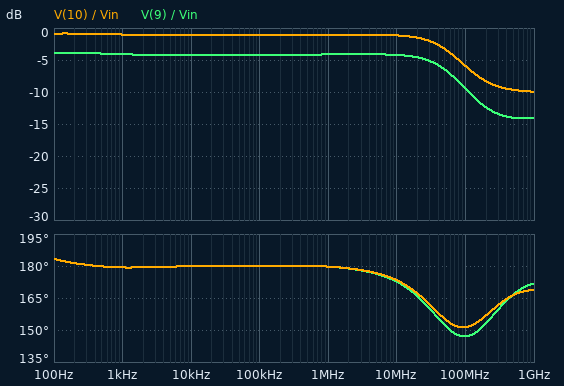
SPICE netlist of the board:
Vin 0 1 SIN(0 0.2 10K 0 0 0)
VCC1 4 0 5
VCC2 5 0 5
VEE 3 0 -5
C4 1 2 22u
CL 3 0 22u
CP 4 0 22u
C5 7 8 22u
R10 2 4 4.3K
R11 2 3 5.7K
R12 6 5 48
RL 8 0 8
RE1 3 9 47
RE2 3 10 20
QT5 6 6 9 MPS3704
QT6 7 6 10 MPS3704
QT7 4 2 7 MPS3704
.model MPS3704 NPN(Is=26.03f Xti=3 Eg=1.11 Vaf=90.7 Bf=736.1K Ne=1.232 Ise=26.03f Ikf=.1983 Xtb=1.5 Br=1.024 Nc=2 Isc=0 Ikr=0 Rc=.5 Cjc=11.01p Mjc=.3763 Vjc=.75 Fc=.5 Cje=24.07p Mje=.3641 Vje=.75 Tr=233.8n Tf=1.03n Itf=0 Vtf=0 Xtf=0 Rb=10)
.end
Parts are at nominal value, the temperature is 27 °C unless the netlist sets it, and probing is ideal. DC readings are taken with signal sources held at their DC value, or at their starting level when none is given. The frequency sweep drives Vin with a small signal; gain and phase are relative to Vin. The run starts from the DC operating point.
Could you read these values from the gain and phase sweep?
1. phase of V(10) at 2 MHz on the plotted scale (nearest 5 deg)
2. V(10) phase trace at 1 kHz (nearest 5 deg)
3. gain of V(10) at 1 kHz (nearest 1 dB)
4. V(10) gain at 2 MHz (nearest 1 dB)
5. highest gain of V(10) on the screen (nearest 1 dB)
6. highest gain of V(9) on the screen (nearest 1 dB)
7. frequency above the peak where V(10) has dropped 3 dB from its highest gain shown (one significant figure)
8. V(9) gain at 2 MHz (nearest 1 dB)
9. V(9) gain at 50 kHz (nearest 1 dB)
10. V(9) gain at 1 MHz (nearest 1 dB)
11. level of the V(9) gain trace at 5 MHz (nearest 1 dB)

180 deg
180 deg
-1 dB
-1 dB
-1 dB
-4 dB
60 MHz
-4 dB
-4 dB
-4 dB
-4 dB
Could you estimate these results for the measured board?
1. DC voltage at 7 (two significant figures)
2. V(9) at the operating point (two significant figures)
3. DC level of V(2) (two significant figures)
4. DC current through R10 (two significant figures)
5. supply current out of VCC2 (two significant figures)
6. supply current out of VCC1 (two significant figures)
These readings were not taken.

-1.7 V
-1.4 V
-930 mV
1.4 mA
120 mA
120 mA
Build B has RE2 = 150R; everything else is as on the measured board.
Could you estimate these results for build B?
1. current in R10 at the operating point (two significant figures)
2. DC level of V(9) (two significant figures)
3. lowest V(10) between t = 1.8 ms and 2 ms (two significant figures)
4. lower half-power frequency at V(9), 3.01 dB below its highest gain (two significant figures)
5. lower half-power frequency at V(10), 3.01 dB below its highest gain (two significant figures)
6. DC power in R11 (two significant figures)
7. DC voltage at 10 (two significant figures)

1.1 mA
-500 mV
-610 mV
5.2 Hz
4.9 Hz
5.0 mW
-490 mV
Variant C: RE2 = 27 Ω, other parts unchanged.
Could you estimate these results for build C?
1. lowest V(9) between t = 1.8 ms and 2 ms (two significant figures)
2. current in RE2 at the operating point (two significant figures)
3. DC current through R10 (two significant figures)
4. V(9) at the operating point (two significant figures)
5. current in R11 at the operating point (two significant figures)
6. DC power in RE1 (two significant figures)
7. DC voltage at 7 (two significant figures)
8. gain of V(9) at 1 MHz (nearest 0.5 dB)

-1.3 V
130 mA
1.3 mA
-1.2 V
770 µA
310 mW
-1.4 V
-4.0 dB
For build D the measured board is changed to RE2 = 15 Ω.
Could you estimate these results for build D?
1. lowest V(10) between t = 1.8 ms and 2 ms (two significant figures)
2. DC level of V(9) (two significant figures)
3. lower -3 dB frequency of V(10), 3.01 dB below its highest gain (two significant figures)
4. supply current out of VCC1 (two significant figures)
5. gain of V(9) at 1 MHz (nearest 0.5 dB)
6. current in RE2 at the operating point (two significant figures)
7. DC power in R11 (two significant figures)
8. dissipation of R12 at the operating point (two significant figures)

-2.3 V
-1.6 V
7.0 Hz
140 mA
-4.0 dB
190 mA
2.5 mW
720 mW
